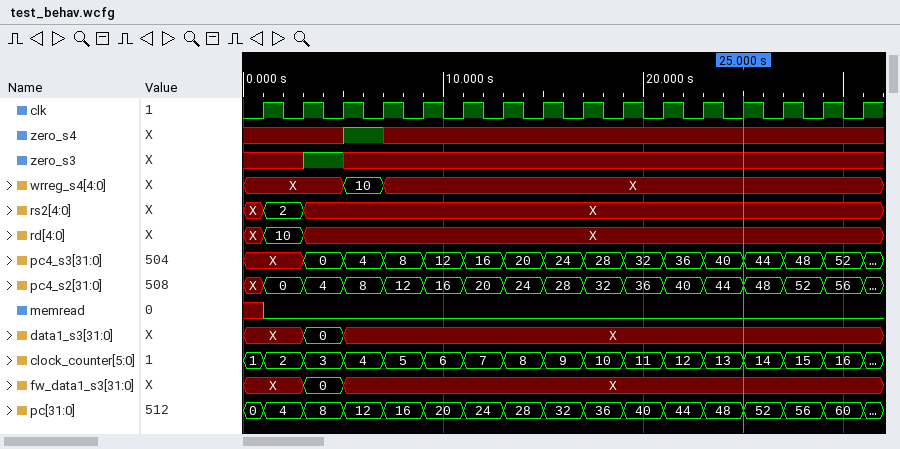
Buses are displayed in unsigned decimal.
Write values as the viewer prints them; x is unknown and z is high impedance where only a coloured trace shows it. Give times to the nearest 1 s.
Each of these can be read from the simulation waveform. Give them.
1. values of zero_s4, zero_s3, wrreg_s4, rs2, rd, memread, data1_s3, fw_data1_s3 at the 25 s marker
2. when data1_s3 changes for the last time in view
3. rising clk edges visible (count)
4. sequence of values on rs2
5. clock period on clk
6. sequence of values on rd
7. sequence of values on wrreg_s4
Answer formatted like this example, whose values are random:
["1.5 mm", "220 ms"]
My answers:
["zero_s4=x, zero_s3=x, wrreg_s4=X, rs2=X, rd=X, memread=0, data1_s3=X, fw_data1_s3=X", "5 s", "16", "X, 2, X", "2 s", "X, 10, X", "X, 10, X"]
